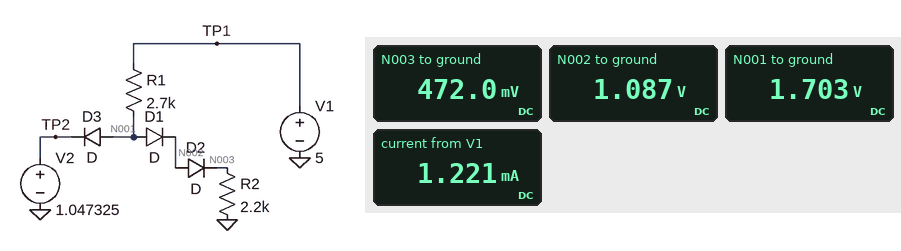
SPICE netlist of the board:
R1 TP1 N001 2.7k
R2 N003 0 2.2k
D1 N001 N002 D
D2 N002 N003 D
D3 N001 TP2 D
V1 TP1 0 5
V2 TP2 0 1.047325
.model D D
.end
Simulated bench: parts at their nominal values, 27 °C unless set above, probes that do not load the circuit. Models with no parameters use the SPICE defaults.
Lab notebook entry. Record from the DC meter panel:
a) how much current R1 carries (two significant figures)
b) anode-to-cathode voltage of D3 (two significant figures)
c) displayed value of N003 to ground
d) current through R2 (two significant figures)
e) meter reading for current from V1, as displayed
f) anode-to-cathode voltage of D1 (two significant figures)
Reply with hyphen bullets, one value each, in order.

- 1.2 mA
- 660 mV
- 472.0 mV
- 210 µA
- 1.221 mA
- 620 mV
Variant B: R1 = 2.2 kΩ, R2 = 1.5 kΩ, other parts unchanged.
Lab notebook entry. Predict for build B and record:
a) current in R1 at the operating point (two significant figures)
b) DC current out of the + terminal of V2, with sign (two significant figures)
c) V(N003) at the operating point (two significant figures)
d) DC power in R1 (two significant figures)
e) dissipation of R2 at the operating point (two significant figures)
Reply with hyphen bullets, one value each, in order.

- 1.5 mA
- -1.2 mA
- 460 mV
- 4.9 mW
- 140 µW
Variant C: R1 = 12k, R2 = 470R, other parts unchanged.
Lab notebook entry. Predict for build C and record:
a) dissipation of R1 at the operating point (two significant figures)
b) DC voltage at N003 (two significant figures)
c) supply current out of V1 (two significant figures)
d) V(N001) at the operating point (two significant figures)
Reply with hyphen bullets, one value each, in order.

- 1.1 mW
- 140 mV
- 300 µA
- 1.4 V
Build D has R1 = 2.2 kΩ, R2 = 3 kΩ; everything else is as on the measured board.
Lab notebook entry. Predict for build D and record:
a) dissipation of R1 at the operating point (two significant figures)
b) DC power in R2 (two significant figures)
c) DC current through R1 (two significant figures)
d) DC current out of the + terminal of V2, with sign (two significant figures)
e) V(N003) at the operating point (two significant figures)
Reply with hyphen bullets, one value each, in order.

- 4.9 mW
- 81 µW
- 1.5 mA
- -1.3 mA
- 490 mV
